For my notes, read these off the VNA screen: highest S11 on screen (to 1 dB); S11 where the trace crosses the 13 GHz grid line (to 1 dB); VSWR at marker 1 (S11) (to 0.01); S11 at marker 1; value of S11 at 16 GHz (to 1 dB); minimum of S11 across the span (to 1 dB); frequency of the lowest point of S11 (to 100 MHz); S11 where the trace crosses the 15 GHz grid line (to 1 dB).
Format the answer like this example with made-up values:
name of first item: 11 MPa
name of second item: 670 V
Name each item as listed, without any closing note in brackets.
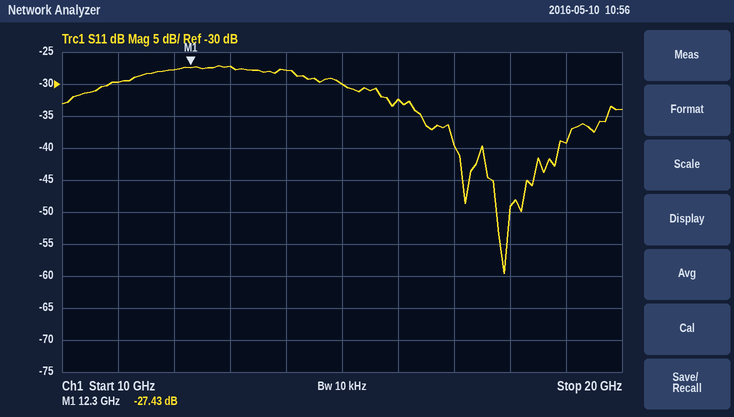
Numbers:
highest S11 on screen: -27 dB
S11 where the trace crosses the 13 GHz grid line: -27 dB
VSWR at marker 1 (S11): 1.09
S11 at marker 1: -27.43 dB
value of S11 at 16 GHz: -32 dB
minimum of S11 across the span: -60 dB
frequency of the lowest point of S11: 17.9 GHz
S11 where the trace crosses the 15 GHz grid line: -30 dB
